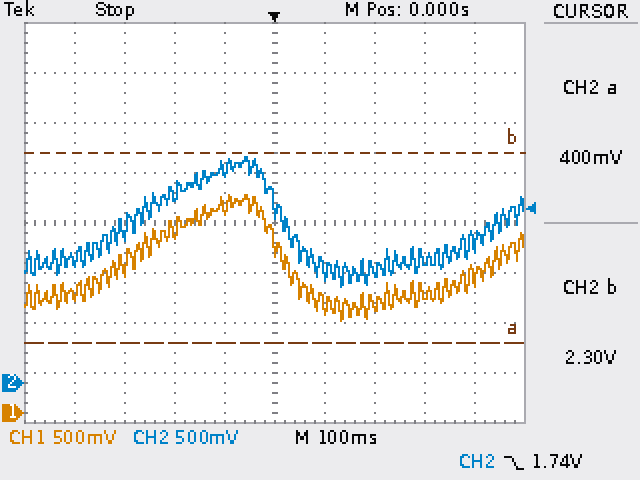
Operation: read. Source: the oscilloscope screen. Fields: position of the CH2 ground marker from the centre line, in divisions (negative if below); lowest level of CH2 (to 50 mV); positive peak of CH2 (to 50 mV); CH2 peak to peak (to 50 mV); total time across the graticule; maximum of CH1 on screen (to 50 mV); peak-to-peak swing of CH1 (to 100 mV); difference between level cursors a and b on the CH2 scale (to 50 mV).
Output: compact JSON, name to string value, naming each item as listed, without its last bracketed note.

{"position of the CH2 ground marker from the centre line, in divisions": "-3.2 div", "lowest level of CH2": "950 mV", "positive peak of CH2": "2.25 V", "CH2 peak to peak": "1.30 V", "total time across the graticule": "1 s", "maximum of CH1 on screen": "2.20 V", "peak-to-peak swing of CH1": "1.30 V", "difference between level cursors a and b on the CH2 scale": "1.90 V"}
